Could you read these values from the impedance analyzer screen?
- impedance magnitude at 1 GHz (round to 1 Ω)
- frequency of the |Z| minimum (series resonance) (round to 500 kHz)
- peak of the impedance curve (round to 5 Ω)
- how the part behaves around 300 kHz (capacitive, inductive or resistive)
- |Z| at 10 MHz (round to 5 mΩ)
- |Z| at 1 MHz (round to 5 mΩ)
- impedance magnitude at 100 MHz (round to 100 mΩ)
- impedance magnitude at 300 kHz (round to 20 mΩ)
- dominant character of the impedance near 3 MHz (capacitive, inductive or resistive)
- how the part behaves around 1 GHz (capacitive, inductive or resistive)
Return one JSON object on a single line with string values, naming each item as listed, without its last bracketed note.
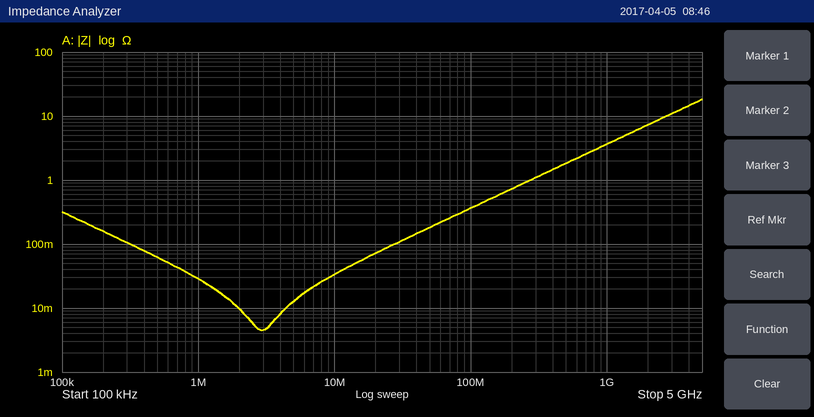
{"impedance magnitude at 1 GHz": "4 Ω", "frequency of the |Z| minimum (series resonance)": "3.0 MHz", "peak of the impedance curve": "20 Ω", "how the part behaves around 300 kHz": "capacitive", "|Z| at 10 MHz": "35 mΩ", "|Z| at 1 MHz": "30 mΩ", "impedance magnitude at 100 MHz": "400 mΩ", "impedance magnitude at 300 kHz": "100 mΩ", "dominant character of the impedance near 3 MHz": "resistive", "how the part behaves around 1 GHz": "inductive"}
